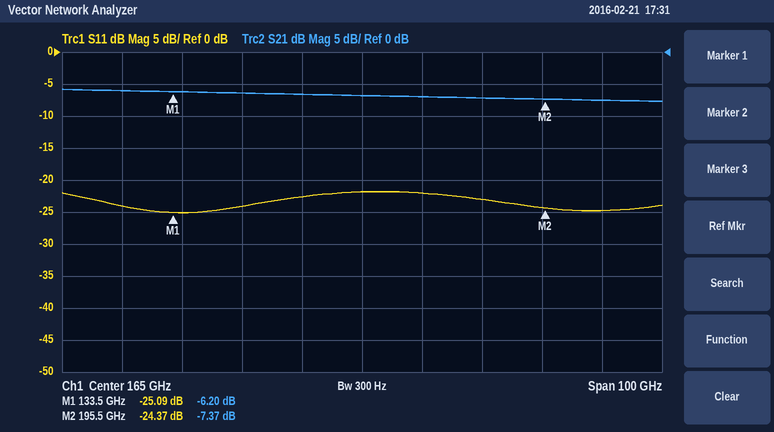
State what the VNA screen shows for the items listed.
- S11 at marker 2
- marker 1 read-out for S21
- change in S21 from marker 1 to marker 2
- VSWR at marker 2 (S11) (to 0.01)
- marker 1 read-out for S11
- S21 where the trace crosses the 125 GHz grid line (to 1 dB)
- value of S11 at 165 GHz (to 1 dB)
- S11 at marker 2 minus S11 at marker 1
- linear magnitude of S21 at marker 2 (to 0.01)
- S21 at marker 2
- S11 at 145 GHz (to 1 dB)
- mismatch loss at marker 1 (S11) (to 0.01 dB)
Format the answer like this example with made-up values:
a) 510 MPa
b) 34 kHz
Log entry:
a) -24.37 dB
b) -6.20 dB
c) -1.17 dB
d) 1.13
e) -25.09 dB
f) -6 dB
g) -22 dB
h) 0.72 dB
i) 0.43
j) -7.37 dB
k) -24 dB
l) 0.01 dB
